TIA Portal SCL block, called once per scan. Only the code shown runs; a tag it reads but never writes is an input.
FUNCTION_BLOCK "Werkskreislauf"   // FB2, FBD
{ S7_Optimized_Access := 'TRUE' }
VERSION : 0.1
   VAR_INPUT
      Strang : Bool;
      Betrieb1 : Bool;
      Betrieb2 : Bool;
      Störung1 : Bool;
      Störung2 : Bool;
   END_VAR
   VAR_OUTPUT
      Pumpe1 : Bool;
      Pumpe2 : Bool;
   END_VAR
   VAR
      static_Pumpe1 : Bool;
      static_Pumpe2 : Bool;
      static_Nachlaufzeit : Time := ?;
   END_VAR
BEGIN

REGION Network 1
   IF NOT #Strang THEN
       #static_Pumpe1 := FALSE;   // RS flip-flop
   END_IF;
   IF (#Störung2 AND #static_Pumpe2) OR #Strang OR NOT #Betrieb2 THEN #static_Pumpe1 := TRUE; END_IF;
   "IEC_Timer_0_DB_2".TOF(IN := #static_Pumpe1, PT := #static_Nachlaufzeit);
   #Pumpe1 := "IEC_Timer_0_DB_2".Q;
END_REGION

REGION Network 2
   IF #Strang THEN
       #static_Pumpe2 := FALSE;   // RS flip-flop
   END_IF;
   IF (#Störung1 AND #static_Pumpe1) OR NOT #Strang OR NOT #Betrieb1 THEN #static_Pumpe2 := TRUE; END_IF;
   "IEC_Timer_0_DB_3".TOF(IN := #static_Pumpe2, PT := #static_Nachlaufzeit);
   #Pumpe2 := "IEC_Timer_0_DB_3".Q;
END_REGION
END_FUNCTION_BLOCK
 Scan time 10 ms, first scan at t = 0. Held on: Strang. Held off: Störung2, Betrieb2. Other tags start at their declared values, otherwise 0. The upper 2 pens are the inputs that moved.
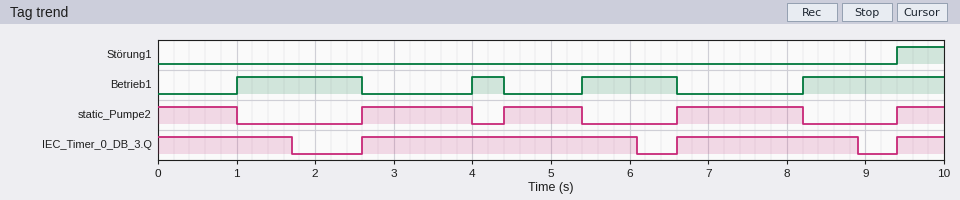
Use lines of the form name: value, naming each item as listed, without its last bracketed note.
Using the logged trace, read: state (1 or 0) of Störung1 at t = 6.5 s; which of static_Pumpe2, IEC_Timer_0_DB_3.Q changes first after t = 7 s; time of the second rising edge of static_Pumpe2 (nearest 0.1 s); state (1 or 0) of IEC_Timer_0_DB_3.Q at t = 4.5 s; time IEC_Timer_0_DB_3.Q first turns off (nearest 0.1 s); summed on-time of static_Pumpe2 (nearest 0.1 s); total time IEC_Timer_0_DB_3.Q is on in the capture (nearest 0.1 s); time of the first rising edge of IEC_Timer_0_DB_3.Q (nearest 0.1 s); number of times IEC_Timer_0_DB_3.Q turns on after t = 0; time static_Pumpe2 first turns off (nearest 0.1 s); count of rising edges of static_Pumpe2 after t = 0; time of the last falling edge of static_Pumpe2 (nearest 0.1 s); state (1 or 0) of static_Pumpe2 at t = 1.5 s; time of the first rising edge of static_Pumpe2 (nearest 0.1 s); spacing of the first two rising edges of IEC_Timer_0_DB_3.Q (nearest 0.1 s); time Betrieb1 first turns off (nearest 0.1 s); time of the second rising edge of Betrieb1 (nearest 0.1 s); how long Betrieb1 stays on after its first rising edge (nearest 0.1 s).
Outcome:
state (1 or 0) of Störung1 at t = 6.5 s: 0
which of static_Pumpe2, IEC_Timer_0_DB_3.Q changes first after t = 7 s: static_Pumpe2
time of the second rising edge of static_Pumpe2: 4.4 s
state (1 or 0) of IEC_Timer_0_DB_3.Q at t = 4.5 s: 1
time IEC_Timer_0_DB_3.Q first turns off: 1.7 s
summed on-time of static_Pumpe2: 5.6 s
total time IEC_Timer_0_DB_3.Q is on in the capture: 8.1 s
time of the first rising edge of IEC_Timer_0_DB_3.Q: 2.6 s
number of times IEC_Timer_0_DB_3.Q turns on after t = 0: 3
time static_Pumpe2 first turns off: 1.0 s
count of rising edges of static_Pumpe2 after t = 0: 4
time of the last falling edge of static_Pumpe2: 8.2 s
state (1 or 0) of static_Pumpe2 at t = 1.5 s: 0
time of the first rising edge of static_Pumpe2: 2.6 s
spacing of the first two rising edges of IEC_Timer_0_DB_3.Q: 4.0 s
time Betrieb1 first turns off: 2.6 s
time of the second rising edge of Betrieb1: 4.0 s
how long Betrieb1 stays on after its first rising edge: 1.6 s
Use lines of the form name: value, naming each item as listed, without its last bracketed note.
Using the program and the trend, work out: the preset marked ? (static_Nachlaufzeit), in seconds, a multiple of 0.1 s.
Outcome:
the preset marked ? (static_Nachlaufzeit), in seconds, a multiple of 0.1 s: 0.7 s
